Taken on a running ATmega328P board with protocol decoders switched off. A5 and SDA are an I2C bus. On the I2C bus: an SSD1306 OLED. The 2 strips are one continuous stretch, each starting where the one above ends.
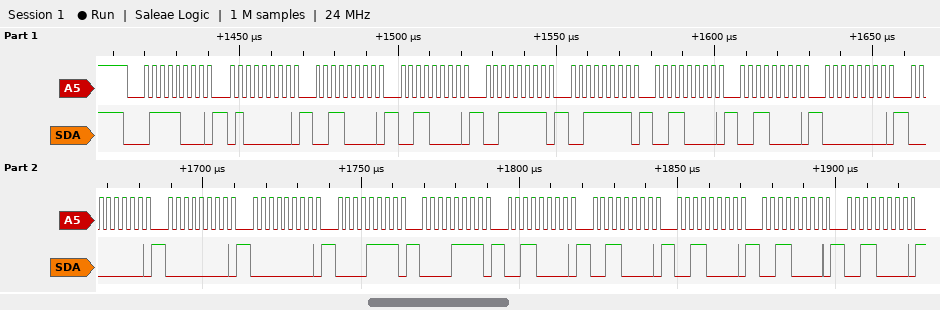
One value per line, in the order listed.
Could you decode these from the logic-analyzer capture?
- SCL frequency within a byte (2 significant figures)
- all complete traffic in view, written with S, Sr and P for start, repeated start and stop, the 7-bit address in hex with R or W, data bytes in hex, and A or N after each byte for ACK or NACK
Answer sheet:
400 kHz
S 3CW A 40 A 30 A 30 A 3F A 3F A 30 A 30 A 00 A 00 A 00 A 00 A 0F A 0F A 30 A 30 A 30 A 30 A 30 A
